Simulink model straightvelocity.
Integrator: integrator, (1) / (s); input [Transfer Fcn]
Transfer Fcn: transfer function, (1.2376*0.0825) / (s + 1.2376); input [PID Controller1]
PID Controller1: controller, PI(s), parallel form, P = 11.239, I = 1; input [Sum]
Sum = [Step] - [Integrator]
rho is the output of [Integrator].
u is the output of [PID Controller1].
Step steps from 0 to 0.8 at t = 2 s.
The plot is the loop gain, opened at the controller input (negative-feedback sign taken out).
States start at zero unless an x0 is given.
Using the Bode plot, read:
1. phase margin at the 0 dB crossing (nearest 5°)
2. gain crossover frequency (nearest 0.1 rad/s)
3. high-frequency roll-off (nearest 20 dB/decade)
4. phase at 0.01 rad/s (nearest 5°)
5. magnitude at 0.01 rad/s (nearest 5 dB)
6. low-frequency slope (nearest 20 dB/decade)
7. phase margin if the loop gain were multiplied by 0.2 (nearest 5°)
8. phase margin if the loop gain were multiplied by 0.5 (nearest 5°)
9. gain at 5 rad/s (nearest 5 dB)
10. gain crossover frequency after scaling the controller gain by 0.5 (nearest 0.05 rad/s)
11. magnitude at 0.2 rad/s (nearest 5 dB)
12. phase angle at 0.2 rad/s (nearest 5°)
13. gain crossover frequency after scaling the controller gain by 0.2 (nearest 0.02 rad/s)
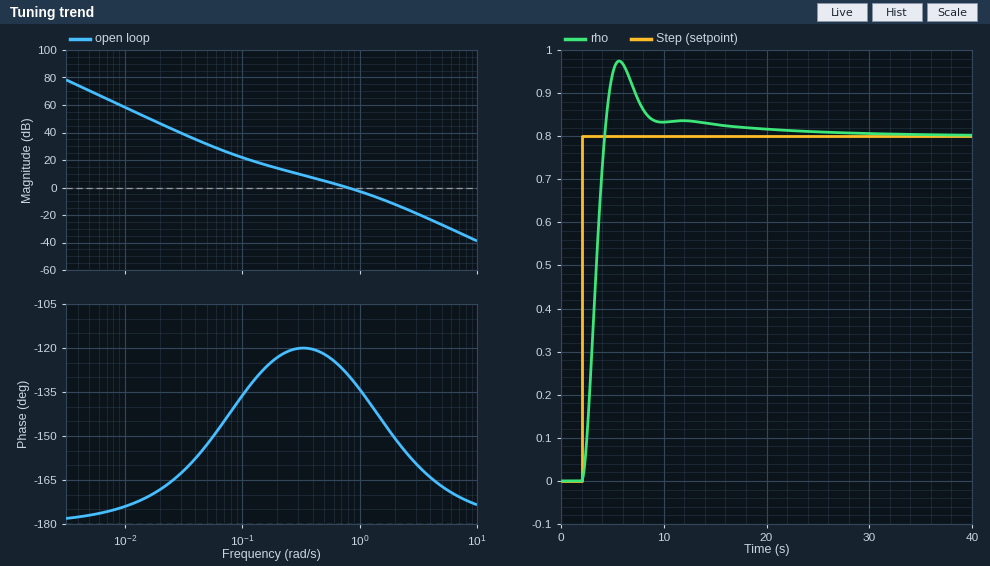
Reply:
50°
0.8 rad/s
-40 dB/decade
-175°
60 dB
-40 dB/decade
55°
60°
-25 dB
0.45 rad/s
15 dB
-125°
0.20 rad/s
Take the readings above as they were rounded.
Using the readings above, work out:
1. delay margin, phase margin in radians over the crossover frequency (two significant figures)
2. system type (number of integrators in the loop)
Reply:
1.1 s
2
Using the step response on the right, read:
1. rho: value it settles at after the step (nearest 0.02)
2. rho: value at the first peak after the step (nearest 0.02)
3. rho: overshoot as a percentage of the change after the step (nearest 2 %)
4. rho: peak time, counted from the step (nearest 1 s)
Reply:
0.80
0.98
22 %
4 s
